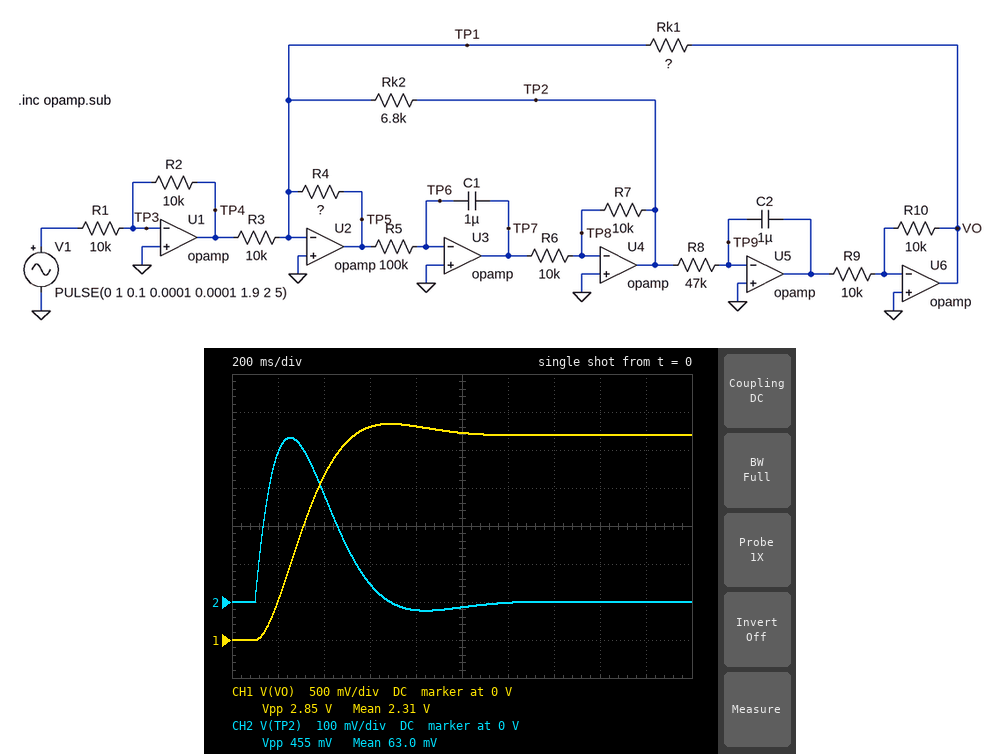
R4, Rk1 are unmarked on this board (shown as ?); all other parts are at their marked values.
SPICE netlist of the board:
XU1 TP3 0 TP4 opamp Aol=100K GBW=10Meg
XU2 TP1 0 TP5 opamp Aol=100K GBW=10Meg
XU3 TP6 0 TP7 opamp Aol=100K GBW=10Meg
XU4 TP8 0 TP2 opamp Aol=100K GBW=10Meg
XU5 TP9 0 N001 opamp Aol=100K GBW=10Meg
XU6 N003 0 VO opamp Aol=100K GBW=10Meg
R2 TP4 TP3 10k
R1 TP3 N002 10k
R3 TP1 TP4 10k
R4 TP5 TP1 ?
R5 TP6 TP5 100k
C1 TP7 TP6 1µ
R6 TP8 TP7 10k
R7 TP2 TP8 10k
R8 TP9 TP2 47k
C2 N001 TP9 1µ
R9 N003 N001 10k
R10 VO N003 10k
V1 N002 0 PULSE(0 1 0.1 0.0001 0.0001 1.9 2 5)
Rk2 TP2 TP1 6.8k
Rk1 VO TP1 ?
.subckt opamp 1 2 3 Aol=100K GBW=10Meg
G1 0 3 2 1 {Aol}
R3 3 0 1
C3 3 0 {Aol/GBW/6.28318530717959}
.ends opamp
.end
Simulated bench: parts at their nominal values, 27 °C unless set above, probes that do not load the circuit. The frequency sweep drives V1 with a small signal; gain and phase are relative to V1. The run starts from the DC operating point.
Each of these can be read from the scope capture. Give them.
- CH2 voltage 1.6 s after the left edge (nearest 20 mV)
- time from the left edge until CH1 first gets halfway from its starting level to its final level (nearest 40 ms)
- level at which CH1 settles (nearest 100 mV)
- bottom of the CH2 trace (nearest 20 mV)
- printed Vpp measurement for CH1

0 V
280 ms
2.7 V
-20 mV
2.85 V
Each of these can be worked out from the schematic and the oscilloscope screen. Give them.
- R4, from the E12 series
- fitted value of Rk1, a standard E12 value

6.8 kΩ
27 kΩ
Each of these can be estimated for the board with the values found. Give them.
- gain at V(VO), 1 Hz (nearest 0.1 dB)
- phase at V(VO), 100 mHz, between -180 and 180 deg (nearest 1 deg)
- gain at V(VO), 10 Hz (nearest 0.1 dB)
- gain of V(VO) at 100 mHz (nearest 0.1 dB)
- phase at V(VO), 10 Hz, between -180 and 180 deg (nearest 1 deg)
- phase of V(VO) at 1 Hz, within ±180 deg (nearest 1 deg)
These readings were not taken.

7.0 dB
-7 deg
-28.7 dB
8.6 dB
-171 deg
-77 deg
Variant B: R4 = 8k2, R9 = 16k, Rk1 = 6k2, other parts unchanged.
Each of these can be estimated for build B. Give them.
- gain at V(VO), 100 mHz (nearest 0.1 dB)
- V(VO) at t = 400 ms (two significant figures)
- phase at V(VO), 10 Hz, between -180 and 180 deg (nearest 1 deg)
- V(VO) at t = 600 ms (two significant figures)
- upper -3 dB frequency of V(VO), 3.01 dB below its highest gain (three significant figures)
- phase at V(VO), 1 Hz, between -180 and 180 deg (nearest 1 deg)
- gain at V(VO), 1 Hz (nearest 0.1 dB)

-4.1 dB
730 mV
-169 deg
600 mV
2.49 Hz
-29 deg
-3.1 dB
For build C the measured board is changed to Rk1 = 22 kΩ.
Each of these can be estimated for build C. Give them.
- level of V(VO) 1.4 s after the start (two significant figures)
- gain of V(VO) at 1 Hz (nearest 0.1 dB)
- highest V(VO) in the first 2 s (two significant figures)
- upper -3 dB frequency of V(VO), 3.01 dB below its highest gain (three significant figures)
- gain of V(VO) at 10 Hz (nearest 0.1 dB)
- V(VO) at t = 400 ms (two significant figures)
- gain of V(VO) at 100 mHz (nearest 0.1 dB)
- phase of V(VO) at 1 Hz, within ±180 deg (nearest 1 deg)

2.2 V
6.5 dB
2.4 V
1.42 Hz
-28.7 dB
2.0 V
6.9 dB
-67 deg
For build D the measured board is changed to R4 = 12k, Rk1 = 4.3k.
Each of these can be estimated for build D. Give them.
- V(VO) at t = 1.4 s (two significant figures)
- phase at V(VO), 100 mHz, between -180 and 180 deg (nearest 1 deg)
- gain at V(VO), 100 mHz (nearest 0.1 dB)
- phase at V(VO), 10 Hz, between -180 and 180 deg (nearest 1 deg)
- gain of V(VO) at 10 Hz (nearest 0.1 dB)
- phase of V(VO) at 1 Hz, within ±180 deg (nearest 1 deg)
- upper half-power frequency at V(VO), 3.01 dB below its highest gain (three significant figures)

430 mV
-1 deg
-7.3 dB
-162 deg
-22.8 dB
-11 deg
4.61 Hz
